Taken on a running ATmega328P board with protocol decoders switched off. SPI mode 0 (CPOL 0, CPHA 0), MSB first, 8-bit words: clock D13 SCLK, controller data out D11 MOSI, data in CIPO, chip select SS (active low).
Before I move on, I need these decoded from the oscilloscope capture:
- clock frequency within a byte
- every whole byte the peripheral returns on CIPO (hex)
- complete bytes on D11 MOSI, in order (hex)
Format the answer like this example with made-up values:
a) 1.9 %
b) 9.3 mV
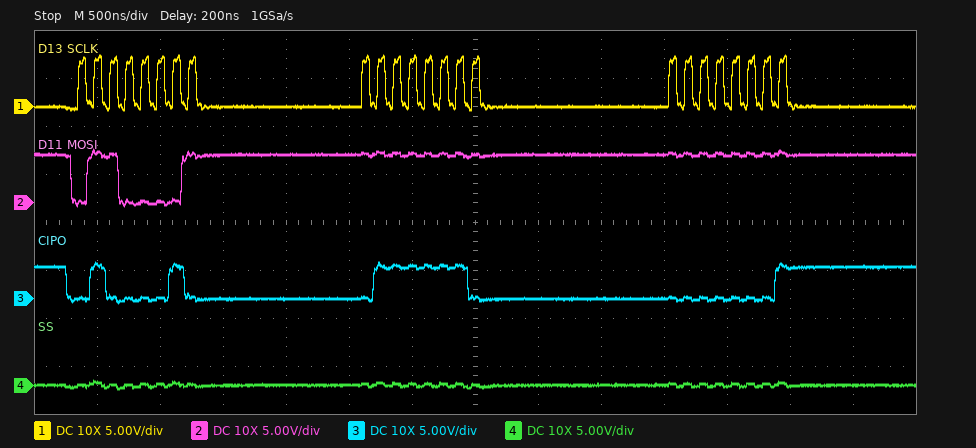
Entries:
a) 8 MHz
b) 42 7E 01
c) 61 FF FF
